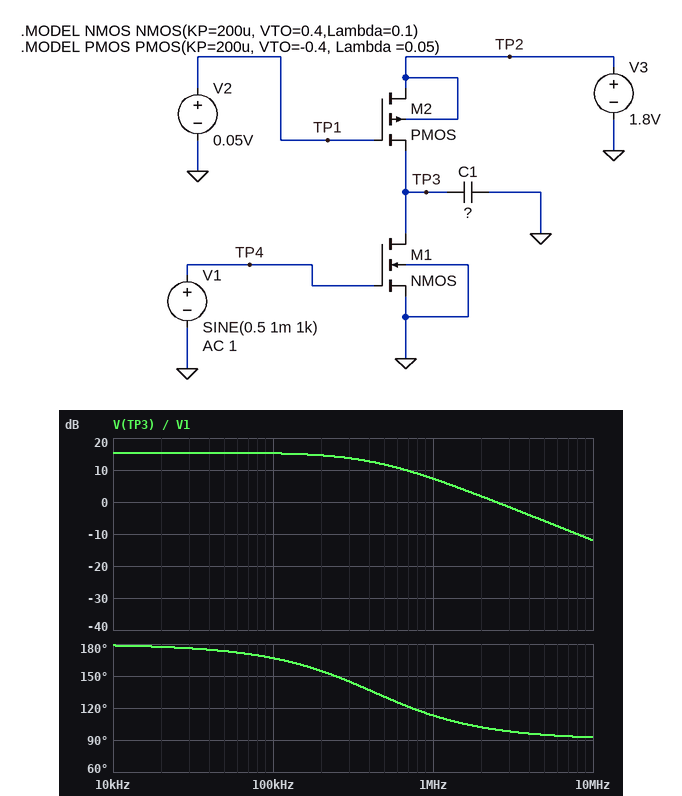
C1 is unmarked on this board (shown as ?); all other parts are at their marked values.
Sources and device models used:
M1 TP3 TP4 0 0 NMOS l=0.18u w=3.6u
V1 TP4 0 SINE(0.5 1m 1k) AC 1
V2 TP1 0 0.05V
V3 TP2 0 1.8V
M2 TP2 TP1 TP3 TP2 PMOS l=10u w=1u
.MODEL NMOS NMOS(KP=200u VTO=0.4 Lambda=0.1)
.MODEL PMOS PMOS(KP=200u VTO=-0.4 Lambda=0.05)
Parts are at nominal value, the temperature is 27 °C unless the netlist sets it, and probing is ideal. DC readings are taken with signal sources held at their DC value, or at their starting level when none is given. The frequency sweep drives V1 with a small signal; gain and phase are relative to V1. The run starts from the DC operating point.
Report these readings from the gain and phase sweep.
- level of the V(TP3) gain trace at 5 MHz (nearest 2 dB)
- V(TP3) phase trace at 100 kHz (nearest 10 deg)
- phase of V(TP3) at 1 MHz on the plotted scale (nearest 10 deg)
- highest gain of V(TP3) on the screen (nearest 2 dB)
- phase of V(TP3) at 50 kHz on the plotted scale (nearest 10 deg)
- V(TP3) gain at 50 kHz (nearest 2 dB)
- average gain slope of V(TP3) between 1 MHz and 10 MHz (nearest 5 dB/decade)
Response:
-6 dB
170 deg
110 deg
16 dB
170 deg
16 dB
-20 dB/decade
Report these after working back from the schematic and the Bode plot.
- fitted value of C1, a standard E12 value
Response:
22 pF
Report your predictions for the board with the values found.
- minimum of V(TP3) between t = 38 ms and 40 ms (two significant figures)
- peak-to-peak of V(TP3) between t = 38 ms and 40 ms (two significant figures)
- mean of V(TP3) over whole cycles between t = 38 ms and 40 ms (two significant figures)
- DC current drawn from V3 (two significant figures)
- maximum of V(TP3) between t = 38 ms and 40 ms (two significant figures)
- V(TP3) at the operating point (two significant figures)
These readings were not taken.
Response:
81 mV
15 mV
87 mV
20 µA
96 mV
86 mV
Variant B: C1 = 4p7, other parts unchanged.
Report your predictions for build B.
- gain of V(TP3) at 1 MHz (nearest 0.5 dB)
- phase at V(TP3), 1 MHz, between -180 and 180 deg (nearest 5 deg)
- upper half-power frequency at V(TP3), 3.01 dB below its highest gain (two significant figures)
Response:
14.5 dB
155 deg
2.0 MHz
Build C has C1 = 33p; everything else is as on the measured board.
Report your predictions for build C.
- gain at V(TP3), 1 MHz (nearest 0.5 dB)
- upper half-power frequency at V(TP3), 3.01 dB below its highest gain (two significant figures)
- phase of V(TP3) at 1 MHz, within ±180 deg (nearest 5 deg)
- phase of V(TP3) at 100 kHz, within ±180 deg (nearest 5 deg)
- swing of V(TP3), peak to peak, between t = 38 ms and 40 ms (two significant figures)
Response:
4.0 dB
280 kHz
105 deg
160 deg
15 mV
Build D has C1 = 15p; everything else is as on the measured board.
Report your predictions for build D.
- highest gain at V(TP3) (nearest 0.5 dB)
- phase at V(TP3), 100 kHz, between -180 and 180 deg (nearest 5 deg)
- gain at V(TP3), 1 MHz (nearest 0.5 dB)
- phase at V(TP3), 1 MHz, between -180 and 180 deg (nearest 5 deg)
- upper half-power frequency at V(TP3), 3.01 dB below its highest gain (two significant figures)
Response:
15.5 dB
170 deg
10.0 dB
120 deg
620 kHz
